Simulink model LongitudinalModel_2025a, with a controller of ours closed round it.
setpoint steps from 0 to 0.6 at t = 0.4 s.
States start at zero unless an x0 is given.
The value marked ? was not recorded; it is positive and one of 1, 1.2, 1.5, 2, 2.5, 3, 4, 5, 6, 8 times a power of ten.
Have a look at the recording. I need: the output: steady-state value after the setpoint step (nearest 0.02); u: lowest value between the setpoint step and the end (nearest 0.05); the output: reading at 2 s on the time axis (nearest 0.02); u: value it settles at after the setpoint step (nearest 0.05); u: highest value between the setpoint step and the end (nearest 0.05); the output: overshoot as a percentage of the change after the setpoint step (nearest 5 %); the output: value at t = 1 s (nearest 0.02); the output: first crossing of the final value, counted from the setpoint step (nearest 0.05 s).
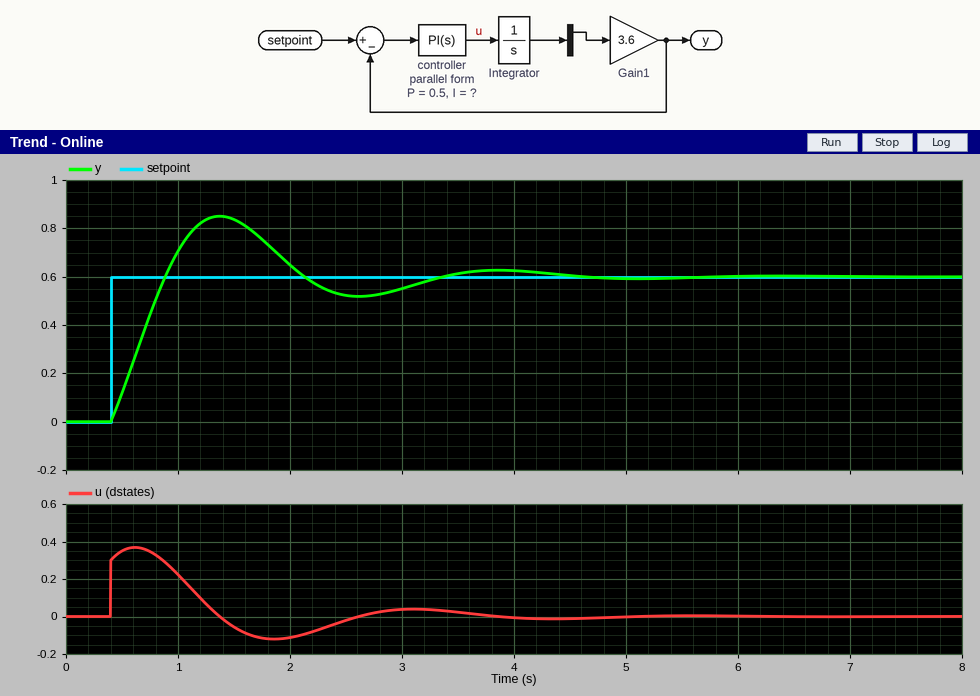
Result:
0.60
-0.10
0.64
0.00
0.35
40 %
0.70
0.50 s
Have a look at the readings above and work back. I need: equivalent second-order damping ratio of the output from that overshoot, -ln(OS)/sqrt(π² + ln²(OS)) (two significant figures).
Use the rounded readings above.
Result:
0.28
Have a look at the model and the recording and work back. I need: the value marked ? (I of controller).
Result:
2
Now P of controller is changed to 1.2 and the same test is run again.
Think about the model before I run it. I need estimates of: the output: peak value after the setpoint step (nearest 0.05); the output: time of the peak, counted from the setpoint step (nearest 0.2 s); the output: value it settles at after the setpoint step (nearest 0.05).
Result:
0.70
0.8 s
0.60
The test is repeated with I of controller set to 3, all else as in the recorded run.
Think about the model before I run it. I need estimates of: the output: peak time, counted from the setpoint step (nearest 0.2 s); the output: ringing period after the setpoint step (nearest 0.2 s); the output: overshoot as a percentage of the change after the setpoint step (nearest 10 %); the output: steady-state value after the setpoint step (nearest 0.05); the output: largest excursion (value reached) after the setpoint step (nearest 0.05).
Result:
0.8 s
2.0 s
50 %
0.60
0.90
